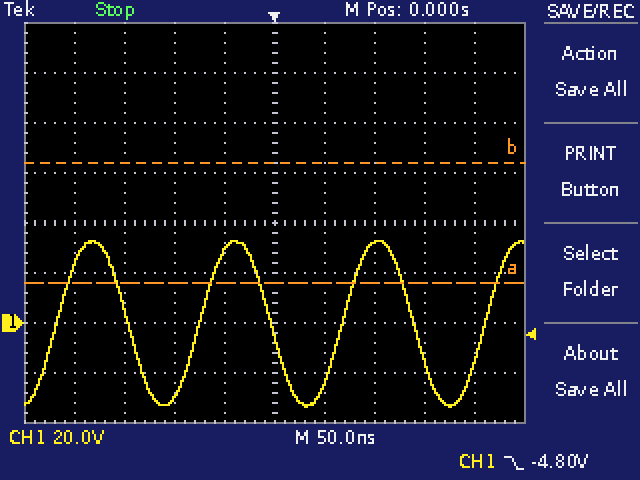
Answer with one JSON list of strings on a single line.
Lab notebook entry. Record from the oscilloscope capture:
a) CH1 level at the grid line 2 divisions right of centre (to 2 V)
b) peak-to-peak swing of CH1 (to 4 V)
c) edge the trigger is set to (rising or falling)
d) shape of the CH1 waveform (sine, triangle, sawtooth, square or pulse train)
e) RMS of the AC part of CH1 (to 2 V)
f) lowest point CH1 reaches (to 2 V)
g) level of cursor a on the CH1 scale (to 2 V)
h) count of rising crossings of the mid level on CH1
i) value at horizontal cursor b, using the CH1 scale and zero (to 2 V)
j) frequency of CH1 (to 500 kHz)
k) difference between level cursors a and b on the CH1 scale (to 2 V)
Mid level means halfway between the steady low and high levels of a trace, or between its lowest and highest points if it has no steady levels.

["32 V", "68 V", "falling", "sine", "24 V", "-34 V", "16 V", "4", "64 V", "7.0 MHz", "48 V"]
